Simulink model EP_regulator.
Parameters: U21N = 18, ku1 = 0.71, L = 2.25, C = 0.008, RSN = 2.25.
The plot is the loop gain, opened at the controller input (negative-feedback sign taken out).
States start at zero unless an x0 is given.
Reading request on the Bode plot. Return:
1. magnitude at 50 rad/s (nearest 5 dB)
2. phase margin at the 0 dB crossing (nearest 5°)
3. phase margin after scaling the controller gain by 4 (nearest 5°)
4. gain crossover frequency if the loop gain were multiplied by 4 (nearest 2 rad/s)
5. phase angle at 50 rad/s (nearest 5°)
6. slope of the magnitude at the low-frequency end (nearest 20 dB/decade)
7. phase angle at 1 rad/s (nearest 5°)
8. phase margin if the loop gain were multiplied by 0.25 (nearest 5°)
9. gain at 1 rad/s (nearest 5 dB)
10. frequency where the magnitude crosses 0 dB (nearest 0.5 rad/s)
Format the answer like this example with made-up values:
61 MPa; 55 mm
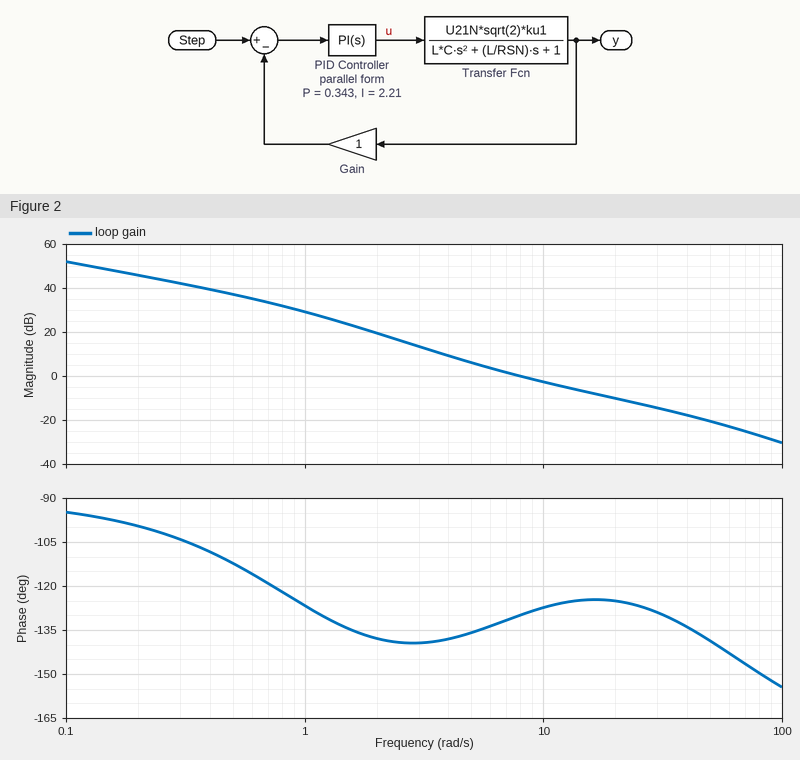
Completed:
-20 dB; 50°; 55°; 24 rad/s; -140°; -20 dB/decade; -125°; 40°; 30 dB; 8.0 rad/s
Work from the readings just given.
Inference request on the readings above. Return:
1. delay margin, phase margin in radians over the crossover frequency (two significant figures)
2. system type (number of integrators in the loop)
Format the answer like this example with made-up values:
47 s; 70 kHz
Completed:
0.11 s; 1
